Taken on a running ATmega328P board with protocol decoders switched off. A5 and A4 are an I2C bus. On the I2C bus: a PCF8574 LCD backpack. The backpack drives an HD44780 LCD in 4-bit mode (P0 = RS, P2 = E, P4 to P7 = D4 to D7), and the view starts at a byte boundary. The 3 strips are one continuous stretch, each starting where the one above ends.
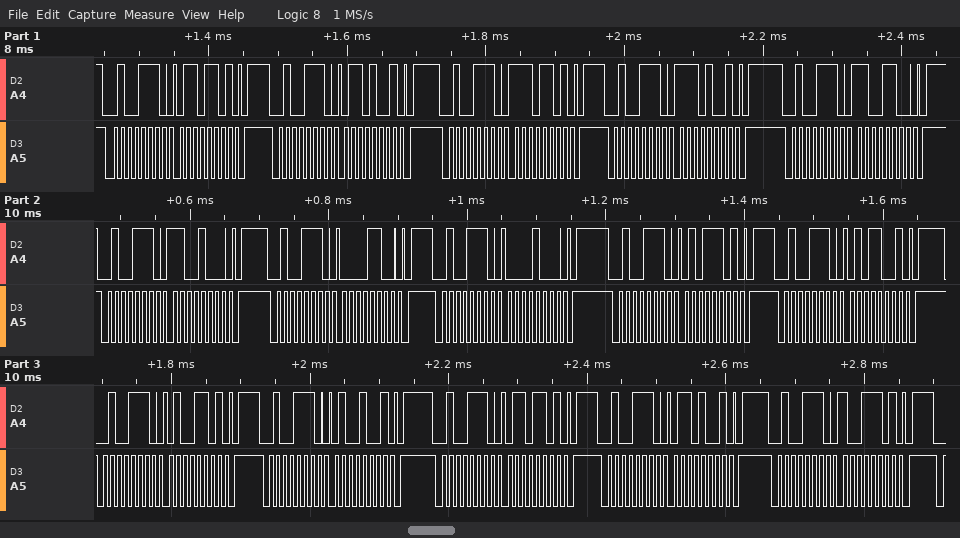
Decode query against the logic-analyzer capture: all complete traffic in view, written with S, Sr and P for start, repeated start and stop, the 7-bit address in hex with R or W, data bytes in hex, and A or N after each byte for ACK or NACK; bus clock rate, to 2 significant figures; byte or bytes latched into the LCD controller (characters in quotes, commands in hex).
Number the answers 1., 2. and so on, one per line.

1. S 27W A 6D A P S 27W A 69 A P S 27W A ED A P S 27W A E9 A P S 27W A CC A P S 27W A C8 A P S 27W A 0C A P S 27W A 08 A P S 27W A 5D A P S 27W A 59 A P S 27W A 4D A P S 27W A 49 A P S 27W A 6D A P S 27W A 69 A P S 27W A 9D A P
2. 100 kHz
3. 'n' 0xC0 'T'
